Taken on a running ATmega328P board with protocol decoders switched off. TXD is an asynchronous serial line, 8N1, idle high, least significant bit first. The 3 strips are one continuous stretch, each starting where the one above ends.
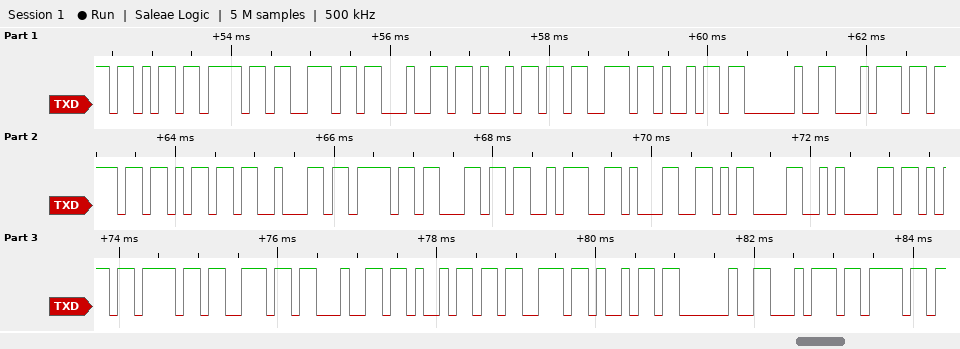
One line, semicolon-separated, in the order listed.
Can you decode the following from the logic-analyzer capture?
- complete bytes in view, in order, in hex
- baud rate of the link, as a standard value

6B 6F 6E 64 69 73 69 20 74 6F 6D 62 6F 6C 3A 31 0D 0A 6B 6F 6E 64 69 73 69 20 74 6F; 9600 baud
